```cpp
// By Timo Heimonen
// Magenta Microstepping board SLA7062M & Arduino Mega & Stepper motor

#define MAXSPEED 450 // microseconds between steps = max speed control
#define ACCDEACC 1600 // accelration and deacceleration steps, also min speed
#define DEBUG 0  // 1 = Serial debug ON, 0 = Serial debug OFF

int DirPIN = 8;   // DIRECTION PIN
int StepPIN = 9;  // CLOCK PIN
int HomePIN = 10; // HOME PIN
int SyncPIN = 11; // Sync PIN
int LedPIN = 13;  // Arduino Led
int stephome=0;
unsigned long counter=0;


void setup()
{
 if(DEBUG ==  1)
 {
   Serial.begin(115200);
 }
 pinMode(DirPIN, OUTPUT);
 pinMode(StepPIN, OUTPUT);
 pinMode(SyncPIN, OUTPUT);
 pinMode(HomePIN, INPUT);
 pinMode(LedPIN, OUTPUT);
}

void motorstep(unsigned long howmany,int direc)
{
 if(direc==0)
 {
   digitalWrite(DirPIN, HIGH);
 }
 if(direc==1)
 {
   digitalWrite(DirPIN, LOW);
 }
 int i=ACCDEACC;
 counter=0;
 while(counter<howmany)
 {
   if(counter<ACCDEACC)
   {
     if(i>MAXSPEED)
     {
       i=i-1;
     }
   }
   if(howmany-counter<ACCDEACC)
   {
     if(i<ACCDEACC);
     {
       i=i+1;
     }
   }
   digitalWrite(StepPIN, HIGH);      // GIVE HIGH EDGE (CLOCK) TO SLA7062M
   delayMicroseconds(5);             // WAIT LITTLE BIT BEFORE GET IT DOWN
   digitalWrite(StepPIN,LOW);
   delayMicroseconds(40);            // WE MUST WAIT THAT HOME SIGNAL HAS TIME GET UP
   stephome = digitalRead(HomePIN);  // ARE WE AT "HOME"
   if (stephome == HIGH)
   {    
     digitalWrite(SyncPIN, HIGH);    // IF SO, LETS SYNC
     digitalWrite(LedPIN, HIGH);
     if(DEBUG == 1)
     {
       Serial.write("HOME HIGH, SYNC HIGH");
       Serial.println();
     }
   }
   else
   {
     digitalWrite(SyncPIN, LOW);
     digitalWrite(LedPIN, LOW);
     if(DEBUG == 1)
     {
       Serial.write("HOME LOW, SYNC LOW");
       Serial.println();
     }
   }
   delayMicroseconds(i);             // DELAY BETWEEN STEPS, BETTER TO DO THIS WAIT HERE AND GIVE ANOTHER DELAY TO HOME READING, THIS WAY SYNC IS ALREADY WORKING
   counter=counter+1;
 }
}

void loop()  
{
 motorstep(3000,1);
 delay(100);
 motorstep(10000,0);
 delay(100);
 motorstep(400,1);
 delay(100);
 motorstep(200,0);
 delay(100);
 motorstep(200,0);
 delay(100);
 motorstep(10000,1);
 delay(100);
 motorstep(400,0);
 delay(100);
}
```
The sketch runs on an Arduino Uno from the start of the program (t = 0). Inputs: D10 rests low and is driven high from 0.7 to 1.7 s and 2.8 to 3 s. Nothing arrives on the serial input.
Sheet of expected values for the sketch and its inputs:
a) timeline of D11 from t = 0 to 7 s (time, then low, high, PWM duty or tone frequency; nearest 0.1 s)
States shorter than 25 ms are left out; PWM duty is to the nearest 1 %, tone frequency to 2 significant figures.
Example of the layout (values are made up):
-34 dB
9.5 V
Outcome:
0 s low; 0.7 s high; 1.7 s low; 2.8 s high; 3 s low
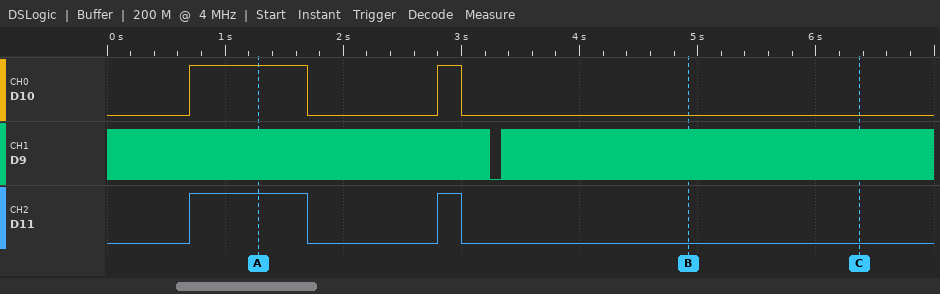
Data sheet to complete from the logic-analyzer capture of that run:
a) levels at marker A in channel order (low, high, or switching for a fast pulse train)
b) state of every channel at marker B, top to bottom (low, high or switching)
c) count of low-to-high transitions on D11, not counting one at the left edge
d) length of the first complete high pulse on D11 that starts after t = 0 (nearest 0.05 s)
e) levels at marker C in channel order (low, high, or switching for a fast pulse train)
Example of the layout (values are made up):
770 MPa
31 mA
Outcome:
D10 high, D9 switching, D11 high
D10 low, D9 switching, D11 low
2
1.00 s
D10 low, D9 switching, D11 low
